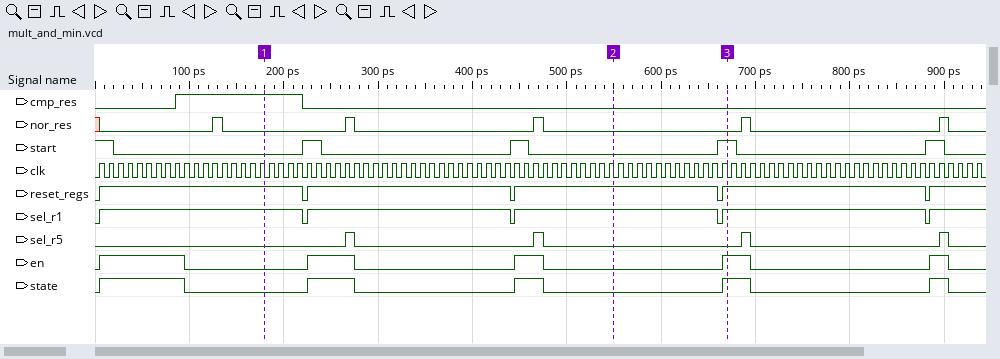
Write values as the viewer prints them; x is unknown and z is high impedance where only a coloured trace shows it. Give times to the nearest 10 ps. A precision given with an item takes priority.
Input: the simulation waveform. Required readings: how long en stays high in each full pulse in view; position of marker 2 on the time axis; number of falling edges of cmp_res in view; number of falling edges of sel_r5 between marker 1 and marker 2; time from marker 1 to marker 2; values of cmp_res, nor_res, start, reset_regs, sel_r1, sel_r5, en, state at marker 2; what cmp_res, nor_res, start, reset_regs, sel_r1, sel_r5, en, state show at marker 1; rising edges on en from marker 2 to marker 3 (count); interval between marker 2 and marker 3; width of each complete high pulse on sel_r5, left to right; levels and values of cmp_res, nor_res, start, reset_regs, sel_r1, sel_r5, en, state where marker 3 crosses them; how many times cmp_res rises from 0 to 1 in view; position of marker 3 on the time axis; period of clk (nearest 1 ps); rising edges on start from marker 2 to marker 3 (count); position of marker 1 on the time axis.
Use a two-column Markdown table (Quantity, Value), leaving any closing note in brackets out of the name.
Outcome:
| Quantity | Value |
|---|---|
| how long en stays high in each full pulse in view | 90 ps, 50 ps, 30 ps, 30 ps, 20 ps |
| position of marker 2 on the time axis | 550 ps |
| number of falling edges of cmp_res in view | 1 |
| number of falling edges of sel_r5 between marker 1 and marker 2 | 2 |
| time from marker 1 to marker 2 | 370 ps |
| values of cmp_res, nor_res, start, reset_regs, sel_r1, sel_r5, en, state at marker 2 | cmp_res=0, nor_res=0, start=0, reset_regs=1, sel_r1=1, sel_r5=0, en=0, state=0 |
| what cmp_res, nor_res, start, reset_regs, sel_r1, sel_r5, en, state show at marker 1 | cmp_res=1, nor_res=0, start=0, reset_regs=1, sel_r1=1, sel_r5=0, en=0, state=0 |
| rising edges on en from marker 2 to marker 3 | 1 |
| interval between marker 2 and marker 3 | 120 ps |
| width of each complete high pulse on sel_r5, left to right | 10 ps, 10 ps, 10 ps, 10 ps |
| levels and values of cmp_res, nor_res, start, reset_regs, sel_r1, sel_r5, en, state where marker 3 crosses them | cmp_res=0, nor_res=0, start=1, reset_regs=1, sel_r1=1, sel_r5=0, en=1, state=1 |
| how many times cmp_res rises from 0 to 1 in view | 1 |
| position of marker 3 on the time axis | 670 ps |
| period of clk | 10 ps |
| rising edges on start from marker 2 to marker 3 | 1 |
| position of marker 1 on the time axis | 180 ps |
